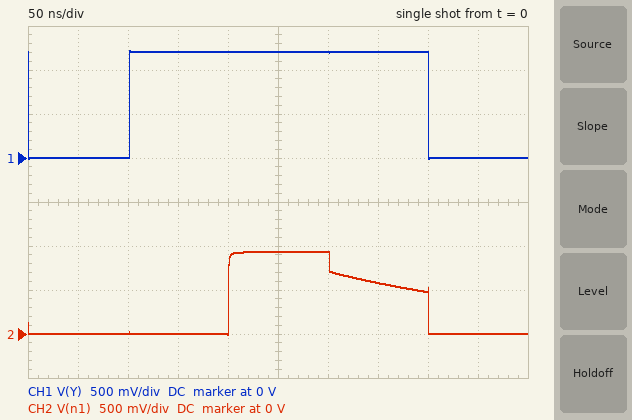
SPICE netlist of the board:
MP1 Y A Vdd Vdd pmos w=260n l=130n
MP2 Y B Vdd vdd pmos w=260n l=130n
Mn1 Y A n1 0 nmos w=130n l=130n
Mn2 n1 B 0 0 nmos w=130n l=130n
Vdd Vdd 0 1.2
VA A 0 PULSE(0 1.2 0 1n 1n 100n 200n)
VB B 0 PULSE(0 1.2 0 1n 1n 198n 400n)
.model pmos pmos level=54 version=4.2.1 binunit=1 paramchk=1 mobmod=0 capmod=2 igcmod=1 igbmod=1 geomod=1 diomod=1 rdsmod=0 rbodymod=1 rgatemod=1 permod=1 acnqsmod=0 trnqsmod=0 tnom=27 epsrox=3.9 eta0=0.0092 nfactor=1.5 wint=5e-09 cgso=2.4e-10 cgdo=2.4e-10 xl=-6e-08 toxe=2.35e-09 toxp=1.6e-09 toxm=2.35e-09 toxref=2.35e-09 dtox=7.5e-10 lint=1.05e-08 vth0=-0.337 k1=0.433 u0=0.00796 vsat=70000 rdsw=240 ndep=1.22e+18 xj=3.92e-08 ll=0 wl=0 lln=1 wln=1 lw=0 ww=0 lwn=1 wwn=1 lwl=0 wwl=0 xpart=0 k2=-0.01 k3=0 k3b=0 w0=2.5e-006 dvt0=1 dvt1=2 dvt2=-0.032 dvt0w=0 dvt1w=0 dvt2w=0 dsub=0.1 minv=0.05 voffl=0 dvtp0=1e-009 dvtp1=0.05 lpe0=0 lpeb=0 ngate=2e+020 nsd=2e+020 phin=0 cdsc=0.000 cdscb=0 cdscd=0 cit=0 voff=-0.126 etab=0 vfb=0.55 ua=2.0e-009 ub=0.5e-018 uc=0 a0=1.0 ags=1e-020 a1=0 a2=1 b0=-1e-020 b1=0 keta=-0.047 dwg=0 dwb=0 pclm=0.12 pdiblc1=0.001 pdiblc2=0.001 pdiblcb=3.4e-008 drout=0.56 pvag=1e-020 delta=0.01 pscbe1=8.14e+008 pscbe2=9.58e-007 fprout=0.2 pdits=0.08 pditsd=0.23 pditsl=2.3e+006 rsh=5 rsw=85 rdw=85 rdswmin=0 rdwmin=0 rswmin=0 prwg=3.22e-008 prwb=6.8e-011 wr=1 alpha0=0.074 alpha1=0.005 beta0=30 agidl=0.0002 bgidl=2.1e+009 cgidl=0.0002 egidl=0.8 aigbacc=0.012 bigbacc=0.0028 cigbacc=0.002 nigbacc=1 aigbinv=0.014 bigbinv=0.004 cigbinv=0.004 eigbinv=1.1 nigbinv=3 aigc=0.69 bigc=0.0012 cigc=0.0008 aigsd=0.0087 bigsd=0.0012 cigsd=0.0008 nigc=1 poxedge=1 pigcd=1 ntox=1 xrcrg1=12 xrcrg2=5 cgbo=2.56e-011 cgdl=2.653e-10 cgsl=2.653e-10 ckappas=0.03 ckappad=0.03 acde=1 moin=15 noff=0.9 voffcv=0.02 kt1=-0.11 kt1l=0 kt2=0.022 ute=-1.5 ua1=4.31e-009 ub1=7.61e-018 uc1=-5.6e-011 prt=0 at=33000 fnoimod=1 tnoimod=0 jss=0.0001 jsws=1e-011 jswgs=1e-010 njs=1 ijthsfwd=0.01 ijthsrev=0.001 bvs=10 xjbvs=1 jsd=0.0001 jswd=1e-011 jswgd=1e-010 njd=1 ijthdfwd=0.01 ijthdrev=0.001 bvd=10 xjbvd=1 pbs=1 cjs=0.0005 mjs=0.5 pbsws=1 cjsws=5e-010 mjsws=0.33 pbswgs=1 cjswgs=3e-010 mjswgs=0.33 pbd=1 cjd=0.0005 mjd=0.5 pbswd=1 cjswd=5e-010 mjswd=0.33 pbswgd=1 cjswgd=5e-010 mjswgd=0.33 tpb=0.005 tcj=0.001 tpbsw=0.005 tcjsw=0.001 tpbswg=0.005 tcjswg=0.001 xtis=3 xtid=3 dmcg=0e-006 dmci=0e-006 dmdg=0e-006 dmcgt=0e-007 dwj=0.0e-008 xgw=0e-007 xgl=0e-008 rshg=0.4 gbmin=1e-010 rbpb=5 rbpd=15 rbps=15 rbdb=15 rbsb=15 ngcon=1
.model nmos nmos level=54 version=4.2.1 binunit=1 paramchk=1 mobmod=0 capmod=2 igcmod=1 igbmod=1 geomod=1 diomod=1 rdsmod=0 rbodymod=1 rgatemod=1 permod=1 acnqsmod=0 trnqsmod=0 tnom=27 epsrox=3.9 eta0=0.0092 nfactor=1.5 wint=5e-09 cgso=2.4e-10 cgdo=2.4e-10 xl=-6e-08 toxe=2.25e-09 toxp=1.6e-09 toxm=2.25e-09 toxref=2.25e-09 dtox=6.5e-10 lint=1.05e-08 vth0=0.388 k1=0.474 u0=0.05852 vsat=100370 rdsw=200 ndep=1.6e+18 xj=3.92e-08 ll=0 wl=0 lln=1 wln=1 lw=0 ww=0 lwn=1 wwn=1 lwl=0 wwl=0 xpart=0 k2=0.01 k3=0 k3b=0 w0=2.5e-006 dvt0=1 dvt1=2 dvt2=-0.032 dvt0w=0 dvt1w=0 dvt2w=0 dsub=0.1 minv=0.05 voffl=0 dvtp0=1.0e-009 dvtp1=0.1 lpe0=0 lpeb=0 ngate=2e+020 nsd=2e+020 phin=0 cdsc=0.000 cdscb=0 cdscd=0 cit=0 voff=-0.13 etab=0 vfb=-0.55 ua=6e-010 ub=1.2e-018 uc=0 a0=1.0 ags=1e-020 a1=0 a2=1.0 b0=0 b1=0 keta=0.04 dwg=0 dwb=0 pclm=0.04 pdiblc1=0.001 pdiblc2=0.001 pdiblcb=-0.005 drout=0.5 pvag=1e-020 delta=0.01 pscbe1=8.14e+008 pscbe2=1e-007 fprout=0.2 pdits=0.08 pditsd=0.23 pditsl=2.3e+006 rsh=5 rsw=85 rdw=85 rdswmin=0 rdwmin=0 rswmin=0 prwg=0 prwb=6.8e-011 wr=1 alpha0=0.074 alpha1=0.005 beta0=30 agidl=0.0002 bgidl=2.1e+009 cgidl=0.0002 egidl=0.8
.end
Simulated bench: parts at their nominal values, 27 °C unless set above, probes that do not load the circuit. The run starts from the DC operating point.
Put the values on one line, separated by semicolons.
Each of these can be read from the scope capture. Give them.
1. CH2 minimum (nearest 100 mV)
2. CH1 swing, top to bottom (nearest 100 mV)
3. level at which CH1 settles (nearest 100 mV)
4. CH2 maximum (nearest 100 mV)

0 V; 1.2 V; 0 V; 900 mV
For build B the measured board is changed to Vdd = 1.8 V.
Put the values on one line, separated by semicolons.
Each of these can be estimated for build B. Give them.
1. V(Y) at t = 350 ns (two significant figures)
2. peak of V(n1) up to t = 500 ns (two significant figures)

1.8 V; 960 mV
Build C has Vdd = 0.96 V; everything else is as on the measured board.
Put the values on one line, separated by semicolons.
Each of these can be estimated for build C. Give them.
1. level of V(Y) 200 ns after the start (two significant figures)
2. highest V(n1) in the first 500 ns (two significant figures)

960 mV; 910 mV
